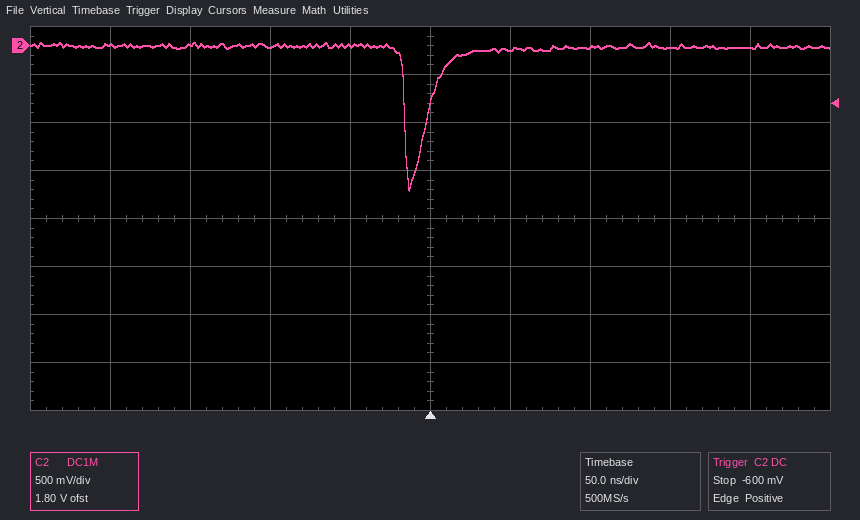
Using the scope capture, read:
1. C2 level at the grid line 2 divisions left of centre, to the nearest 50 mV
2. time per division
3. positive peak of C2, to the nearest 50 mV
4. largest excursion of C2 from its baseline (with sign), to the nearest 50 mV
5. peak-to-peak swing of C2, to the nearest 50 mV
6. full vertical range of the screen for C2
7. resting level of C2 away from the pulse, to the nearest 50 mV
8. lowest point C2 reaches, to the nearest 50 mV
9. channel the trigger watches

0 mV
50 ns
50 mV
-1.50 V
1.55 V
4 V
0 mV
-1.50 V
C2
